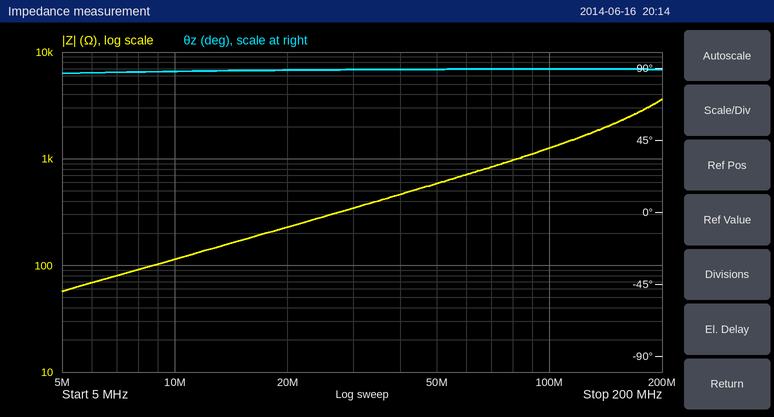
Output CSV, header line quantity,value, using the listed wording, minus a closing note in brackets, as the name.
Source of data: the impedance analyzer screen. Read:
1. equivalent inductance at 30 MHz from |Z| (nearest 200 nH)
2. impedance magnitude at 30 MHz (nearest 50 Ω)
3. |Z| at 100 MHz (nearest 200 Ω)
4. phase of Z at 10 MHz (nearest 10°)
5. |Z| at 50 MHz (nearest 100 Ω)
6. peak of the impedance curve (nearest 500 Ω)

quantity,value
equivalent inductance at 30 MHz from |Z|,1.8 µH
impedance magnitude at 30 MHz,350 Ω
|Z| at 100 MHz,1.2 kΩ
phase of Z at 10 MHz,90°
|Z| at 50 MHz,600 Ω
peak of the impedance curve,3.5 kΩ
